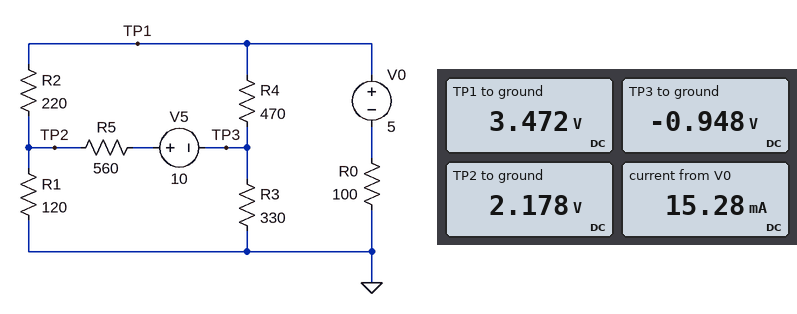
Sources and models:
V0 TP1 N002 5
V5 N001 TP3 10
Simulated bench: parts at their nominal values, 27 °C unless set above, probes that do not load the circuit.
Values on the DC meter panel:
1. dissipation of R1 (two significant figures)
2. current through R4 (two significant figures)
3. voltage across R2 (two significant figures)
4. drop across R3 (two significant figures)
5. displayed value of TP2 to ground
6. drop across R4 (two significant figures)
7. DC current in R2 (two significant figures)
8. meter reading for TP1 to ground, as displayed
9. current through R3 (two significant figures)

40 mW
9.4 mA
1.3 V
950 mV
2.178 V
4.4 V
5.9 mA
3.472 V
2.9 mA
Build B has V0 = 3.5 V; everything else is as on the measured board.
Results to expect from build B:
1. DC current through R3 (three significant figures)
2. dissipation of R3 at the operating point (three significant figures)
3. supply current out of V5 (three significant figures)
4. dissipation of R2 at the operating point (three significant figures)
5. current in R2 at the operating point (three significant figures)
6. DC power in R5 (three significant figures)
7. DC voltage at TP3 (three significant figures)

4.15 mA
5.68 mW
12.2 mA
1.72 mW
2.80 mA
83.3 mW
-1.37 V
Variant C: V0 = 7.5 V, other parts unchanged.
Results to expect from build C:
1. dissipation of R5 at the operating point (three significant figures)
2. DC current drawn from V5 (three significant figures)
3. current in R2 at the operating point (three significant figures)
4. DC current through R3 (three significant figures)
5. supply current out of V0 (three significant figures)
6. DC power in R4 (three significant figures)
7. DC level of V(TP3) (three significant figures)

86.1 mW
12.4 mA
11.0 mA
744 µA
22.7 mA
63.9 mW
-246 mV
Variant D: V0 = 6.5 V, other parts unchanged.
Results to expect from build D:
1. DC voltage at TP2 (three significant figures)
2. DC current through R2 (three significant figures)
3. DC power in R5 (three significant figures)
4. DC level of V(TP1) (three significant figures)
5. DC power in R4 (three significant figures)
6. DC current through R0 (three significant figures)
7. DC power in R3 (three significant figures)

2.56 V
8.96 mA
85.4 mW
4.53 V
54.4 mW
19.7 mA
840 µW
